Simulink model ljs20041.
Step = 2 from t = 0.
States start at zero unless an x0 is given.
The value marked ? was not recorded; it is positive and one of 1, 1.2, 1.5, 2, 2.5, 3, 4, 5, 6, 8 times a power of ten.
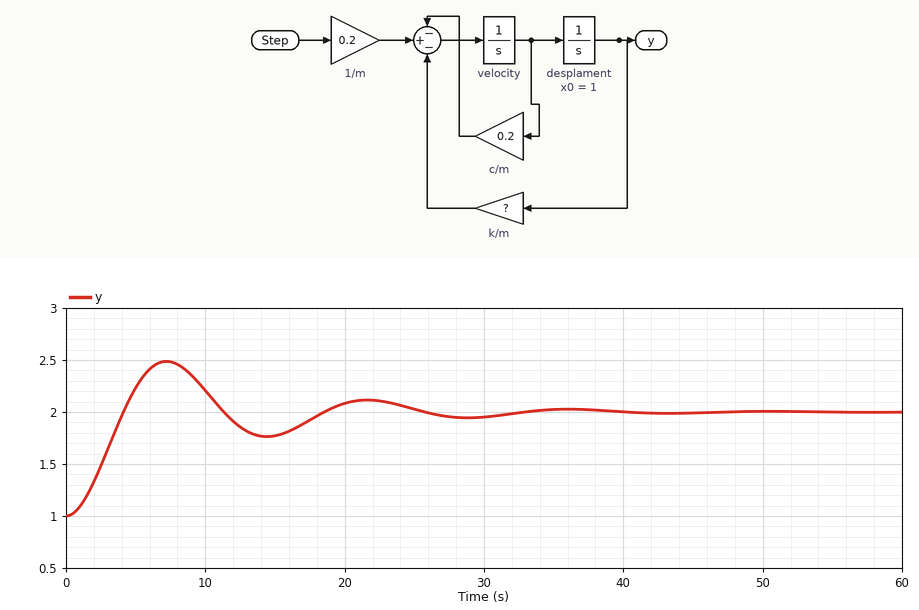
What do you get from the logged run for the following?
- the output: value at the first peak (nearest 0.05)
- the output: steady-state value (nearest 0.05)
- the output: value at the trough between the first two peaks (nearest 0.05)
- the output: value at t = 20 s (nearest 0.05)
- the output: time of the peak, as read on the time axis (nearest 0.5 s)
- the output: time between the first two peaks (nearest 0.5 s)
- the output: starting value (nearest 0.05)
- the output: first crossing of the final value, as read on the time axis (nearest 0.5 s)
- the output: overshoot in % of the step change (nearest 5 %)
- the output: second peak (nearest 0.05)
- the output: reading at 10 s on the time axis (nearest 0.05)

2.50
2.00
1.75
2.10
7.0 s
14.5 s
1.00
4.0 s
50 %
2.10
2.20
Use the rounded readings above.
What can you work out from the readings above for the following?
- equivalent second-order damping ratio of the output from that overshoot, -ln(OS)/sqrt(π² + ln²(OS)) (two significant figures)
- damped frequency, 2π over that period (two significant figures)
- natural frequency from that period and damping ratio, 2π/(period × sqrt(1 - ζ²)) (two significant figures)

0.22
0.43 rad/s
0.44 rad/s
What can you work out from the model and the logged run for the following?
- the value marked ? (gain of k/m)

0.2
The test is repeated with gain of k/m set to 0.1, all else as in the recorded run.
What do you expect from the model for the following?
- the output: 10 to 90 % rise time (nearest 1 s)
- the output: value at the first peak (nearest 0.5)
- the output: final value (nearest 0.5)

4 s
5.0
4.0
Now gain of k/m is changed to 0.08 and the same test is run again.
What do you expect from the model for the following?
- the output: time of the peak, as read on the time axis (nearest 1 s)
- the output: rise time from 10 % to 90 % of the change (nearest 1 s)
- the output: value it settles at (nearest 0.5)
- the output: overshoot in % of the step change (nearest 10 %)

12 s
5 s
5.0
30 %
